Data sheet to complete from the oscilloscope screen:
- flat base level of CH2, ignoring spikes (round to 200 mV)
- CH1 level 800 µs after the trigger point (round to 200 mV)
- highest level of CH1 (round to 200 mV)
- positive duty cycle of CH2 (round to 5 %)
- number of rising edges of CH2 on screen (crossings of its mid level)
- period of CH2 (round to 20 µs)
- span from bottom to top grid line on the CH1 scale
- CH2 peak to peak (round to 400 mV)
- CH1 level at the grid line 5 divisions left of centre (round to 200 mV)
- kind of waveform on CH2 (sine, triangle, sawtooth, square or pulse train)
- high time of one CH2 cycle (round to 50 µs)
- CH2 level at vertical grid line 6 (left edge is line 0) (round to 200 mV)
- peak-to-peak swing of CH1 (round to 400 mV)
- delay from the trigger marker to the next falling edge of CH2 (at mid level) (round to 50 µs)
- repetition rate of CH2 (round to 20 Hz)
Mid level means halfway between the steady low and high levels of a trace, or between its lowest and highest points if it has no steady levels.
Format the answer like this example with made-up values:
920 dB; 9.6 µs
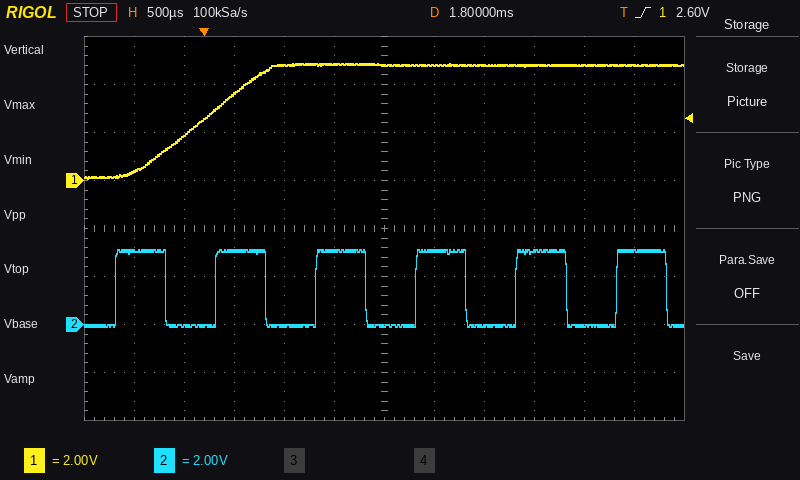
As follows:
0.0 V; 4.8 V; 4.8 V; 50 %; 6; 1.00 ms; 16 V; 3.2 V; 400 mV; square; 500 µs; 0.0 V; 4.8 V; 600 µs; 1.00 kHz
